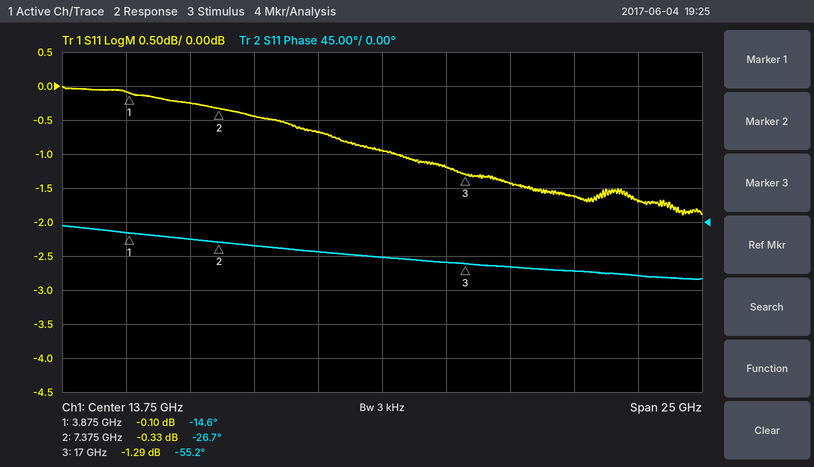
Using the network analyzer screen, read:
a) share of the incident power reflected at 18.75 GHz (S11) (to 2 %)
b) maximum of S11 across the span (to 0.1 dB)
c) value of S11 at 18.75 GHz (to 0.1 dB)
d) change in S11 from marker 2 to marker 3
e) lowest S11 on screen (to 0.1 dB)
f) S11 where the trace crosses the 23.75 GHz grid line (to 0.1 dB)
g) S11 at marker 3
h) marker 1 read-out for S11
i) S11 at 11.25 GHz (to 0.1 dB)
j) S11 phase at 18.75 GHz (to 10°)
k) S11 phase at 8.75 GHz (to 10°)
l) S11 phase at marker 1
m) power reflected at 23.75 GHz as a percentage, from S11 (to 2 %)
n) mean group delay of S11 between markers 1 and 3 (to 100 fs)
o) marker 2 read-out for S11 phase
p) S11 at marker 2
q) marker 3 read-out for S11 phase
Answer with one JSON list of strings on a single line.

["72 %", "0.0 dB", "-1.4 dB", "-0.96 dB", "-1.9 dB", "-1.7 dB", "-1.29 dB", "-0.10 dB", "-0.7 dB", "-60°", "-30°", "-14.6°", "68 %", "8.6 ps", "-26.7°", "-0.33 dB", "-55.2°"]
